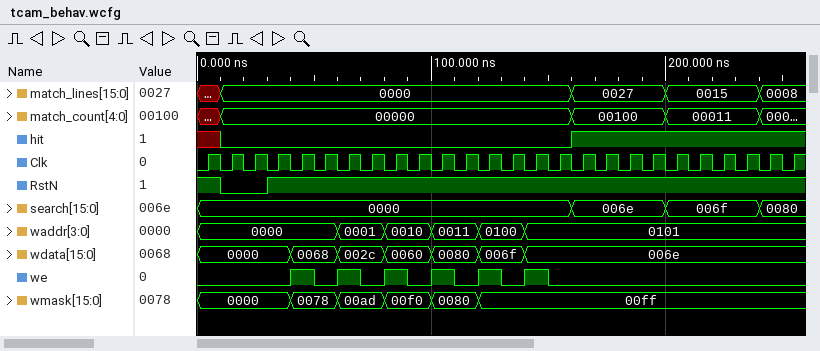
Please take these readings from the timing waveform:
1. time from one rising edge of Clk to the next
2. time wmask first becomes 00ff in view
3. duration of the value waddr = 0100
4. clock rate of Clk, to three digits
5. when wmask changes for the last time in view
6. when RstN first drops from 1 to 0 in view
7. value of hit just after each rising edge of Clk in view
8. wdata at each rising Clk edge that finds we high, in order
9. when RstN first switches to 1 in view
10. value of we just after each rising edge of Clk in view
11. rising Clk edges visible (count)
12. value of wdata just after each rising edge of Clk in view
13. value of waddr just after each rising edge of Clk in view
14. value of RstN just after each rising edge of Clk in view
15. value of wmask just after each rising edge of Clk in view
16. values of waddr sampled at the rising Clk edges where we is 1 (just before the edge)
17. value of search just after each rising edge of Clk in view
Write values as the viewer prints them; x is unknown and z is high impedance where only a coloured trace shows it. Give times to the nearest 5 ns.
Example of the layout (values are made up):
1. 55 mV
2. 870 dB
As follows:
1. 10 ns
2. 120 ns
3. 20 ns
4. 100 MHz
5. 120 ns
6. 10 ns
7. x 0 0 0 0 0 0 0 0 0 0 0 0 0 0 0 1 1 1 1 1 1 1 1 1 1
8. 0068, 002c, 0060, 0080, 006f, 006e
9. 30 ns
10. 0 0 0 0 1 0 1 0 1 0 1 0 1 0 1 0 0 0 0 0 0 0 0 0 0 0
11. 26
12. 0000, 0000, 0000, 0000, 0068, 0068, 002c, 002c, 0060, 0060, 0080, 0080, 006f, 006f, 006e, 006e, 006e, 006e, 006e, 006e, 006e, 006e, 006e, 006e, 006e, 006e
13. 0000, 0000, 0000, 0000, 0000, 0000, 0001, 0001, 0010, 0010, 0011, 0011, 0100, 0100, 0101, 0101, 0101, 0101, 0101, 0101, 0101, 0101, 0101, 0101, 0101, 0101
14. 1 0 0 1 1 1 1 1 1 1 1 1 1 1 1 1 1 1 1 1 1 1 1 1 1 1
15. 0000, 0000, 0000, 0000, 0078, 0078, 00ad, 00ad, 00f0, 00f0, 0080, 0080, 00ff, 00ff, 00ff, 00ff, 00ff, 00ff, 00ff, 00ff, 00ff, 00ff, 00ff, 00ff, 00ff, 00ff
16. 0000, 0001, 0010, 0011, 0100, 0101
17. 0000, 0000, 0000, 0000, 0000, 0000, 0000, 0000, 0000, 0000, 0000, 0000, 0000, 0000, 0000, 0000, 006e, 006e, 006e, 006e, 006f, 006f, 006f, 006f, 0080, 0080
